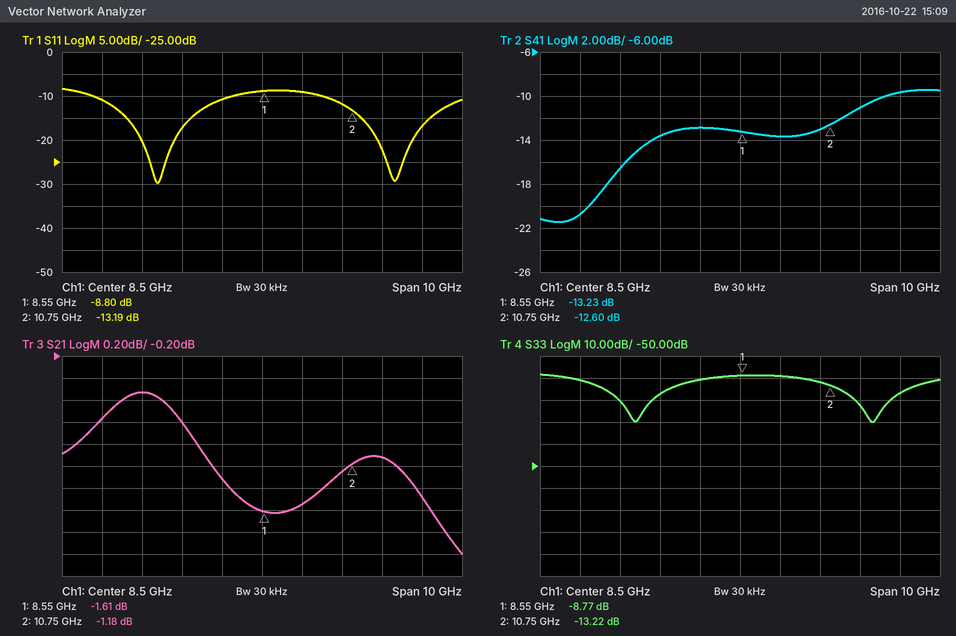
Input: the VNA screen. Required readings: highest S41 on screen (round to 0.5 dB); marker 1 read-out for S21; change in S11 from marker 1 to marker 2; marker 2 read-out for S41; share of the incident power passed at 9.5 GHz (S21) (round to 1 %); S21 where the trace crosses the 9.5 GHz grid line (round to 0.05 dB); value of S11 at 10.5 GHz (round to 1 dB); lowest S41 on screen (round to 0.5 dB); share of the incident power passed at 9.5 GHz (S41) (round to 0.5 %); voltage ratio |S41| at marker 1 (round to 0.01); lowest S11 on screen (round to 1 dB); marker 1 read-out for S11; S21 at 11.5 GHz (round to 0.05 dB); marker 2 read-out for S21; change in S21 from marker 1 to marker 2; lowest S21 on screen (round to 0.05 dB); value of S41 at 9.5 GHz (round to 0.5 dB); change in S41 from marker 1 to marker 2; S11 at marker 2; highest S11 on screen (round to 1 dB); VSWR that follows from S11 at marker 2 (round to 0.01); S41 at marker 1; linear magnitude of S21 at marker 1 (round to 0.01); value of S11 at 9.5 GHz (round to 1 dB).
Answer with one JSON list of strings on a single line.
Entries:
["-9.5 dB", "-1.61 dB", "-4.39 dB", "-12.60 dB", "70 %", "-1.55 dB", "-12 dB", "-21.5 dB", "4.5 %", "0.22", "-30 dB", "-8.80 dB", "-1.10 dB", "-1.18 dB", "0.43 dB", "-2.00 dB", "-13.5 dB", "0.63 dB", "-13.19 dB", "-8 dB", "1.56", "-13.23 dB", "0.83", "-9 dB"]
